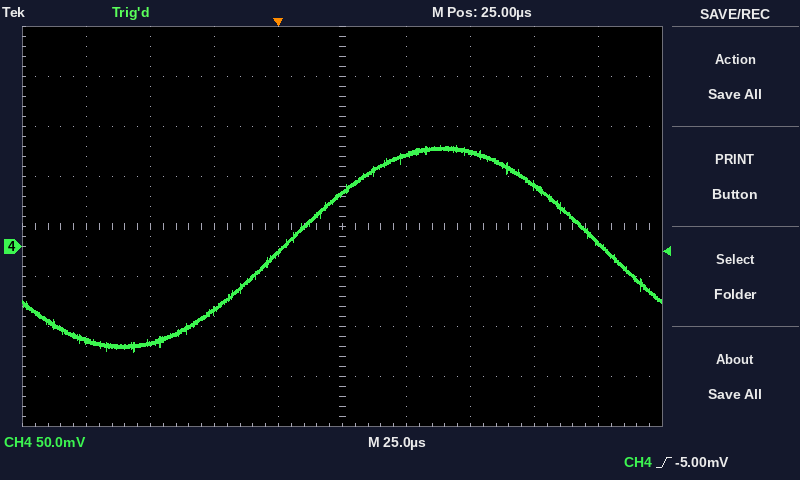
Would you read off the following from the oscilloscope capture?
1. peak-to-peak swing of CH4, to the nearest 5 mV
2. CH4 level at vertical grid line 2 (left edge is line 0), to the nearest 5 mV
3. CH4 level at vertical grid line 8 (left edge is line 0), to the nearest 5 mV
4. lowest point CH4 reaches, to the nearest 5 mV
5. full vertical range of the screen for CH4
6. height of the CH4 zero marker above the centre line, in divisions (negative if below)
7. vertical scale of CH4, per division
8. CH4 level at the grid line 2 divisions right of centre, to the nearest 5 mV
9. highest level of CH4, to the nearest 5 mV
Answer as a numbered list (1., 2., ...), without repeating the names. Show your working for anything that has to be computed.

1. 100 mV − (-105 mV) = 205 mV
2. -95 mV
3. 60 mV
4. -105 mV
5. 400 mV
6. -0.4 div
7. 50 mV
8. 95 mV
9. 100 mV
